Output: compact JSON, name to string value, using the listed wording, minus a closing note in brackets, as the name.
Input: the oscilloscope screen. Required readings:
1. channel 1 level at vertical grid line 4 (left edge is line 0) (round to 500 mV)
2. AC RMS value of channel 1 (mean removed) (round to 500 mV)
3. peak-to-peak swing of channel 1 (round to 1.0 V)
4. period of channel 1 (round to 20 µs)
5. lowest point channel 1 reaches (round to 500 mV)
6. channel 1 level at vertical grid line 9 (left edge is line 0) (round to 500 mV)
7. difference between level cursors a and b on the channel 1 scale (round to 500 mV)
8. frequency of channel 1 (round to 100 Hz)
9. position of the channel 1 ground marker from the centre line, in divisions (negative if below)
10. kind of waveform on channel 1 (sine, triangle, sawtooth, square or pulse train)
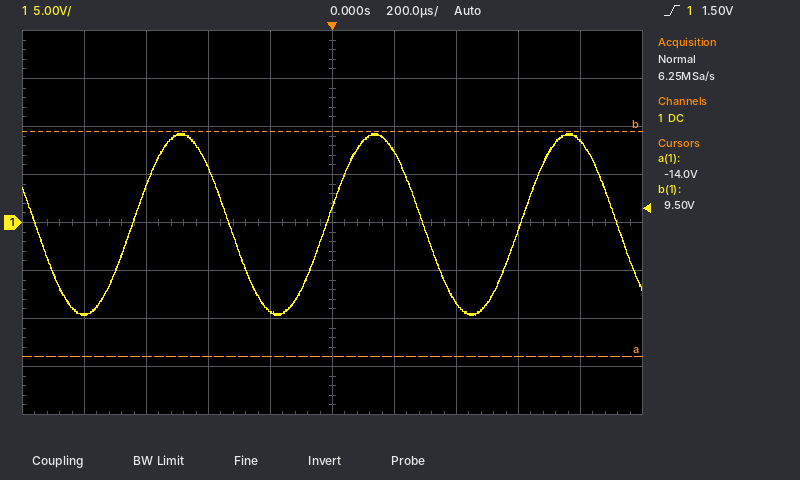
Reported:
{"channel 1 level at vertical grid line 4 (left edge is line 0)": "-9.0 V", "AC RMS value of channel 1 (mean removed)": "6.5 V", "peak-to-peak swing of channel 1": "19.0 V", "period of channel 1": "620 µs", "lowest point channel 1 reaches": "-9.5 V", "channel 1 level at vertical grid line 9 (left edge is line 0)": "8.5 V", "difference between level cursors a and b on the channel 1 scale": "23.5 V", "frequency of channel 1": "1.6 kHz", "position of the channel 1 ground marker from the centre line, in divisions": "0.0 div", "kind of waveform on channel 1": "sine"}
